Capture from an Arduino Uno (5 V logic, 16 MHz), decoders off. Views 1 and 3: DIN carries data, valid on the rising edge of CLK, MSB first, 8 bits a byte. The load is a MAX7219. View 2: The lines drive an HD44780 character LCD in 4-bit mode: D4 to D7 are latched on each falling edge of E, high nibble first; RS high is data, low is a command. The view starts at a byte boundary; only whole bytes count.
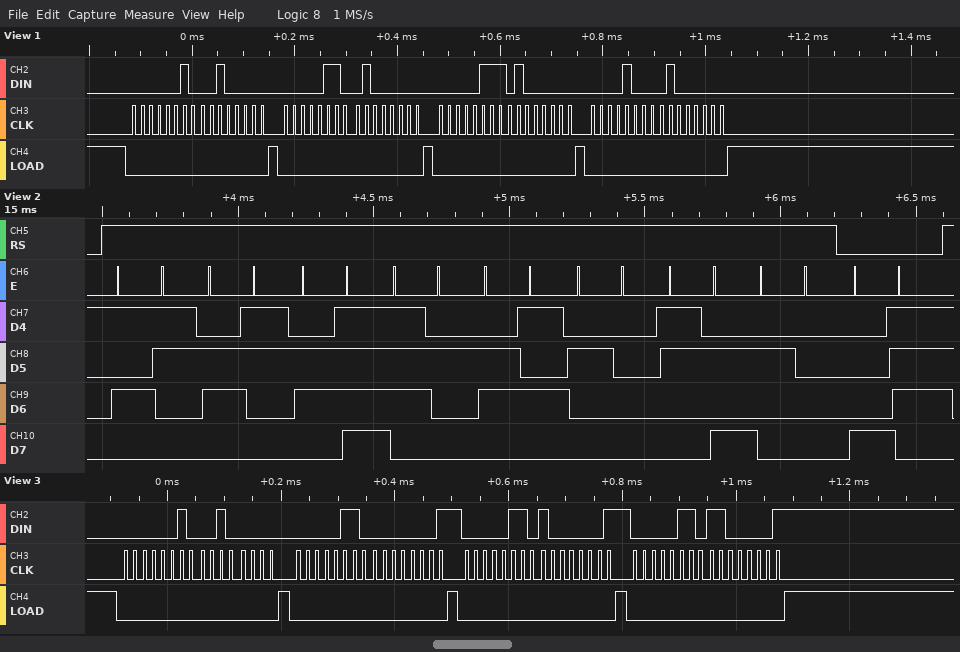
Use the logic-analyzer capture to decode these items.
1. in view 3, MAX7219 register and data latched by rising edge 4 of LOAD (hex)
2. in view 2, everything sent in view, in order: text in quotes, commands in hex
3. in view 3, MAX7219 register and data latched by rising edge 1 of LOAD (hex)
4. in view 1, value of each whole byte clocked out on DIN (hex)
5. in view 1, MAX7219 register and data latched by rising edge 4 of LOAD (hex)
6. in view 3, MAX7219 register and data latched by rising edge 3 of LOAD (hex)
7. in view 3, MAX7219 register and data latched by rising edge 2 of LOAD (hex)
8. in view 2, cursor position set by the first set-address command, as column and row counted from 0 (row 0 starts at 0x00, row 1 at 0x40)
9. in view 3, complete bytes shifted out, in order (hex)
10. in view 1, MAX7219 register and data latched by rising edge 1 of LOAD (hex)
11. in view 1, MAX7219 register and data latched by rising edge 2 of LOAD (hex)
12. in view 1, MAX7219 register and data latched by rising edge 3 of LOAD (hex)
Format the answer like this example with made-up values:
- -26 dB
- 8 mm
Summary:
- register 0x6, data 0xC1
- "Score : " 0x87
- register 0x2, data 0x20
- 0x02 0x20 0x06 0x40 0x07 0x40 0x08 0x40
- register 0x8, data 0x40
- register 0x6, data 0x81
- register 0x6, data 0x01
- column 7, row 0
- 02 20 06 01 06 81 06 C1
- register 0x2, data 0x20
- register 0x6, data 0x40
- register 0x7, data 0x40
